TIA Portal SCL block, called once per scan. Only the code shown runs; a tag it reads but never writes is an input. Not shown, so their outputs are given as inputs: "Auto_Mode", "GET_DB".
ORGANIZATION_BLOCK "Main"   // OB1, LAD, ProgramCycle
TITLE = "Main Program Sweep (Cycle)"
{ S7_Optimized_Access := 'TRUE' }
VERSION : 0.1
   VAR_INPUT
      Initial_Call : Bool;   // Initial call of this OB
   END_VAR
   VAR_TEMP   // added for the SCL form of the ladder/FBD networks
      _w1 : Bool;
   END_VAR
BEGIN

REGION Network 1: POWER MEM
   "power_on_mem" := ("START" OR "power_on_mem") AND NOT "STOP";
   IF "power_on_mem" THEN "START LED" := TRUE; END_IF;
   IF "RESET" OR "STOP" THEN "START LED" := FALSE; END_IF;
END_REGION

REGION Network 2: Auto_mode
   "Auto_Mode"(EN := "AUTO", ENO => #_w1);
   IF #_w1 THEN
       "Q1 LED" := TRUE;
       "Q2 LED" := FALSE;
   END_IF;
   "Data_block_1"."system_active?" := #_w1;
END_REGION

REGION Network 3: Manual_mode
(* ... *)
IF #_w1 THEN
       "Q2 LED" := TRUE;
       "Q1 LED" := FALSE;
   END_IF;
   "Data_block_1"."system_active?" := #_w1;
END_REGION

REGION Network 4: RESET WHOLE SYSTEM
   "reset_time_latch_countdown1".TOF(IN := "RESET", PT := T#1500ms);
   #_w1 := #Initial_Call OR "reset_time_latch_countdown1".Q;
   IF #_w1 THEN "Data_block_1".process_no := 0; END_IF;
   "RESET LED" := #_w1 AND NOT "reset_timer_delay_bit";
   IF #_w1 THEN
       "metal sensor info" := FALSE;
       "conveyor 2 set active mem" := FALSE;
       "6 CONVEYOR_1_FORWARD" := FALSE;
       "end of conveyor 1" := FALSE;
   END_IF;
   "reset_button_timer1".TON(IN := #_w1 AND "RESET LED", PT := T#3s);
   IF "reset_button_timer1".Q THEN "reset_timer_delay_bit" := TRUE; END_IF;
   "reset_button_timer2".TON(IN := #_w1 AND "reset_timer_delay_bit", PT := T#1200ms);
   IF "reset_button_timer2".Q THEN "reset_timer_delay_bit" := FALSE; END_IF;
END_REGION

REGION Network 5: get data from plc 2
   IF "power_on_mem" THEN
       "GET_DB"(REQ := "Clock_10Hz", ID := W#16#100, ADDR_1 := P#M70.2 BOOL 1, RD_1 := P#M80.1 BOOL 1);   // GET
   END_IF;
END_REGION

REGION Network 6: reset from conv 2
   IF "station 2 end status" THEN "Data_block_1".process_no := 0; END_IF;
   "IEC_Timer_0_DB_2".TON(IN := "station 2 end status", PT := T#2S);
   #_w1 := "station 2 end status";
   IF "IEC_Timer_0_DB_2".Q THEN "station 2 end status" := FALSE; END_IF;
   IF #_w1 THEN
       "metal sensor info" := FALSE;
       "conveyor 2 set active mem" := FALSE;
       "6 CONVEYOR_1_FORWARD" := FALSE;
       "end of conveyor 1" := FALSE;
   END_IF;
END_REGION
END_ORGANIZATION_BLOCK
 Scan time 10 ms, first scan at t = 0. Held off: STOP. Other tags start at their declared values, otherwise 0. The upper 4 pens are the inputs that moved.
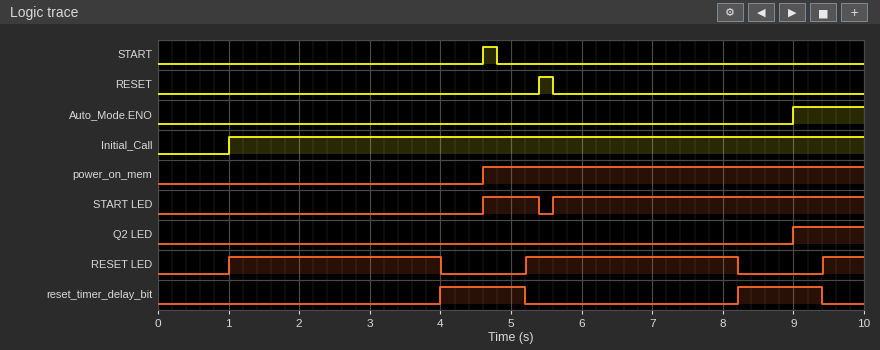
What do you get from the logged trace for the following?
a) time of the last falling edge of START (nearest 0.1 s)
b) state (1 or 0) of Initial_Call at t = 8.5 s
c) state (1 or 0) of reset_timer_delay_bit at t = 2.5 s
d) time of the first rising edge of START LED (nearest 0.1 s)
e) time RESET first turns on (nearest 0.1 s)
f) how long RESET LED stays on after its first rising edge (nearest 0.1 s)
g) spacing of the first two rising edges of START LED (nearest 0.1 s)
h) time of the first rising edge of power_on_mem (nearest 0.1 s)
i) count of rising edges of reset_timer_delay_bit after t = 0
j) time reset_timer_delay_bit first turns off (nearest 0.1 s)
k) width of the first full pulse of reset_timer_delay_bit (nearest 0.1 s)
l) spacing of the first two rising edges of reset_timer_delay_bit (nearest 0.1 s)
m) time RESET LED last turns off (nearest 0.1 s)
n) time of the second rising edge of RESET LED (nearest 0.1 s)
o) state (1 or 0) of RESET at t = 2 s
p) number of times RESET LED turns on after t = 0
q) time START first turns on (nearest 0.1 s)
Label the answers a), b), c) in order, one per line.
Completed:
a) 4.8 s
b) 1
c) 0
d) 4.6 s
e) 5.4 s
f) 3.0 s
g) 1.0 s
h) 4.6 s
i) 2
j) 5.2 s
k) 1.2 s
l) 4.2 s
m) 8.2 s
n) 5.2 s
o) 0
p) 3
q) 4.6 s
